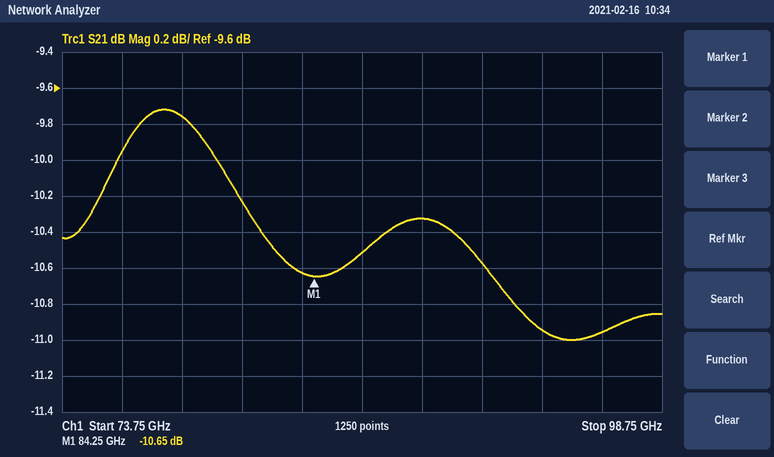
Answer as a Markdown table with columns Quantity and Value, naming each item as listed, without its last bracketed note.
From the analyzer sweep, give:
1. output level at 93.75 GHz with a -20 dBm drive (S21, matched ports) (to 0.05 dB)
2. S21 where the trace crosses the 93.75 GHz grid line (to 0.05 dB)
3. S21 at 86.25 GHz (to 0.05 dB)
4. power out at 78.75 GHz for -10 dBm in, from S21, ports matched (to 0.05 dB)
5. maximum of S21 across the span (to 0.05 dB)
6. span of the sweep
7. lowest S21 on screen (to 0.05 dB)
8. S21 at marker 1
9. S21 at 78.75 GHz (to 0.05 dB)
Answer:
| Quantity | Value |
|---|---|
| output level at 93.75 GHz with a -20 dBm drive (S21, matched ports) | -30.95 dBm |
| S21 where the trace crosses the 93.75 GHz grid line | -10.95 dB |
| S21 at 86.25 GHz | -10.50 dB |
| power out at 78.75 GHz for -10 dBm in, from S21, ports matched | -19.75 dBm |
| maximum of S21 across the span | -9.70 dB |
| span of the sweep | 25 GHz |
| lowest S21 on screen | -11.00 dB |
| S21 at marker 1 | -10.65 dB |
| S21 at 78.75 GHz | -9.75 dB |
